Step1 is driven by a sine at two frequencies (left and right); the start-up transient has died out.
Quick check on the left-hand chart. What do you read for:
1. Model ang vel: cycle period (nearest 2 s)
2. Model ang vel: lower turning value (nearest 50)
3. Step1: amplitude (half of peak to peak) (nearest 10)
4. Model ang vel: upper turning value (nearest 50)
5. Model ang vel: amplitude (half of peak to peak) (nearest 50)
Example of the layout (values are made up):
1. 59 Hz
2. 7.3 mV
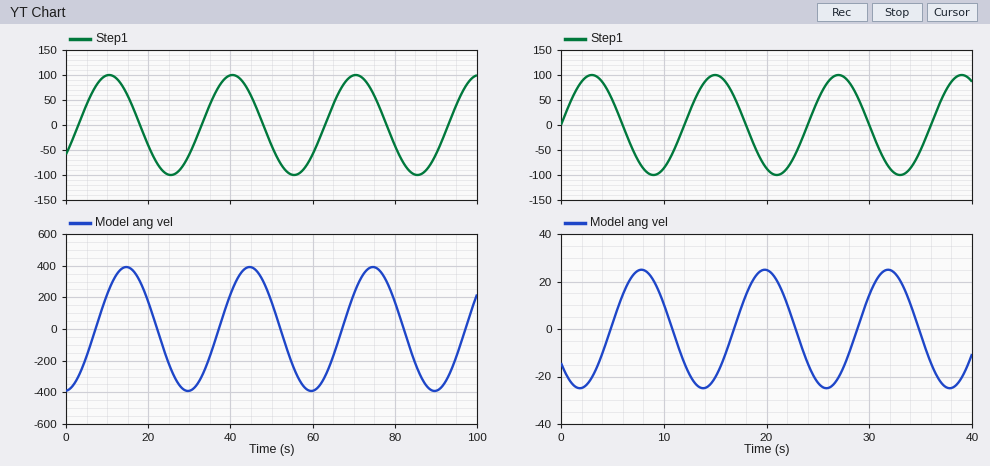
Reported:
1. 30 s
2. -400
3. 100
4. 400
5. 400
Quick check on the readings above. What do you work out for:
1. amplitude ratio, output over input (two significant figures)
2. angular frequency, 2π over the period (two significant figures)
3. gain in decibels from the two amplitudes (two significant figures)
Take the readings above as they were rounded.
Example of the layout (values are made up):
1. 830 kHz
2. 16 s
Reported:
1. 4.0
2. 0.21 rad/s
3. 12 dB
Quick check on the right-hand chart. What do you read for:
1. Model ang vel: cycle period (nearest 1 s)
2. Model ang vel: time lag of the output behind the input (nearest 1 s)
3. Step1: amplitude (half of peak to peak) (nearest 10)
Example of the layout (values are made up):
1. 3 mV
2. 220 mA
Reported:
1. 12 s
2. 5 s
3. 100
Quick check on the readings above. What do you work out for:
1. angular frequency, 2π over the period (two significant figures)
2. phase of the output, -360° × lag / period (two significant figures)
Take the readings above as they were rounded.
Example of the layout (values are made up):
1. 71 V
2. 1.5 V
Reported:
1. 0.52 rad/s
2. -150°
